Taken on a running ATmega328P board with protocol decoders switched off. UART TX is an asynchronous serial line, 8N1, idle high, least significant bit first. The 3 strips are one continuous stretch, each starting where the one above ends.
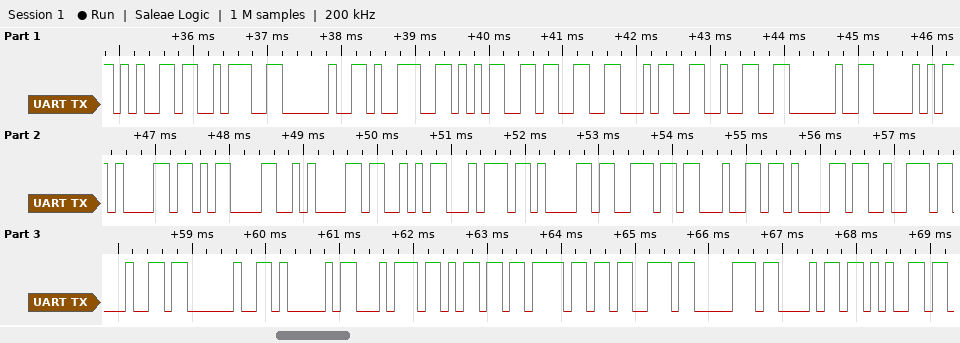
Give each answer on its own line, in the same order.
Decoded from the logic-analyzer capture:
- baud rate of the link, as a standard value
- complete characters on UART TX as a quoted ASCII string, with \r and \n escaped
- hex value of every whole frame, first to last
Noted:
9600 baud
"e: 95342 Pa\r\nStandard Atmosphe"
65 3A 20 39 35 33 34 32 20 50 61 0D 0A 53 74 61 6E 64 61 72 64 20 41 74 6D 6F 73 70 68 65
